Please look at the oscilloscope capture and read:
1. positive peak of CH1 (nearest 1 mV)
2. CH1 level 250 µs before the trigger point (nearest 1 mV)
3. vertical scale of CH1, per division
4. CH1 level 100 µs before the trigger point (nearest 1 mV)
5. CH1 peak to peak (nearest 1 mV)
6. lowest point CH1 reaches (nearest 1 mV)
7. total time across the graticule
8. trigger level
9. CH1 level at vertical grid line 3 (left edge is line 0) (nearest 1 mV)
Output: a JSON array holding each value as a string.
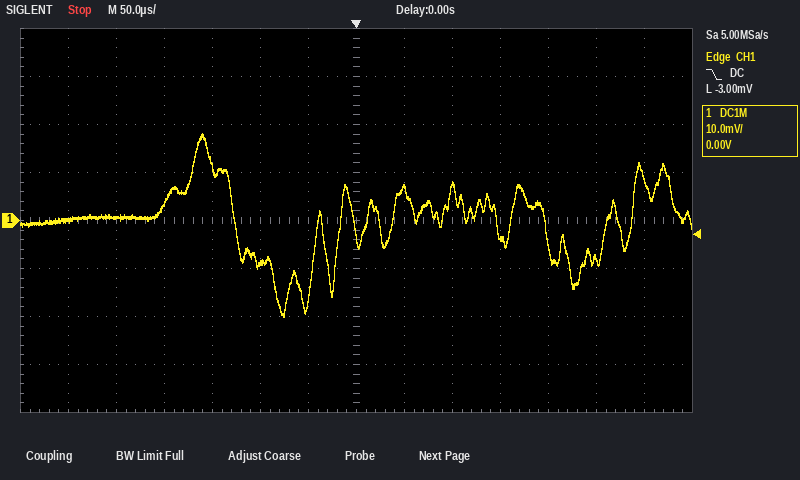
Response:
["18 mV", "1 mV", "10 mV", "-9 mV", "38 mV", "-20 mV", "700 µs", "-3.00 mV", "4 mV"]
